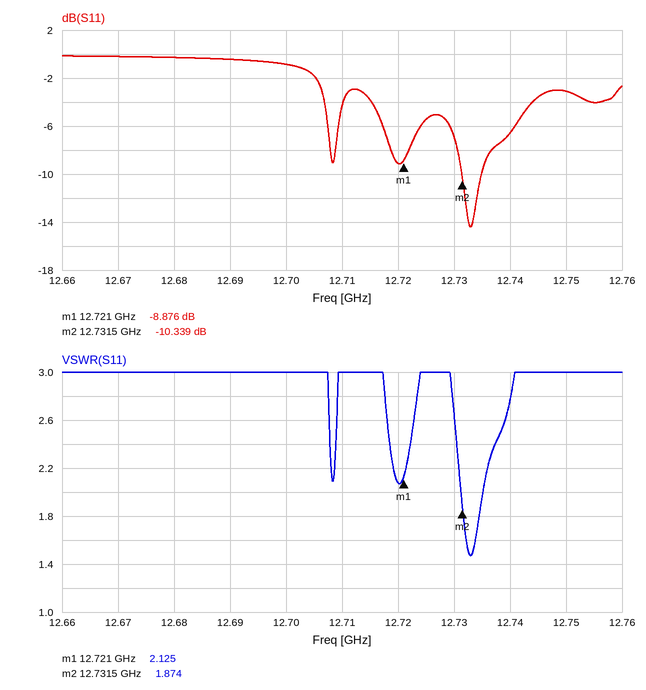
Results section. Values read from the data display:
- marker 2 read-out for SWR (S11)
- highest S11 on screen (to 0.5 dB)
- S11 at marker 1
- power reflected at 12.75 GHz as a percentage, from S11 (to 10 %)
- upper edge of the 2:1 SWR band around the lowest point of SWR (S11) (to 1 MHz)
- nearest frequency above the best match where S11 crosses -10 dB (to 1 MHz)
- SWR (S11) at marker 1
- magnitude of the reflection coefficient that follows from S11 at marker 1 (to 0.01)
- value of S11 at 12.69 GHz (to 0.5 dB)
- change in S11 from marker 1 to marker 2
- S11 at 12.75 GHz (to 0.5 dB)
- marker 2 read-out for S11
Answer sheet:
1.874
0.0 dB
-8.876 dB
50 %
12.735 GHz
12.735 GHz
2.125
0.36
-0.5 dB
-1.463 dB
-3.0 dB
-10.339 dB
